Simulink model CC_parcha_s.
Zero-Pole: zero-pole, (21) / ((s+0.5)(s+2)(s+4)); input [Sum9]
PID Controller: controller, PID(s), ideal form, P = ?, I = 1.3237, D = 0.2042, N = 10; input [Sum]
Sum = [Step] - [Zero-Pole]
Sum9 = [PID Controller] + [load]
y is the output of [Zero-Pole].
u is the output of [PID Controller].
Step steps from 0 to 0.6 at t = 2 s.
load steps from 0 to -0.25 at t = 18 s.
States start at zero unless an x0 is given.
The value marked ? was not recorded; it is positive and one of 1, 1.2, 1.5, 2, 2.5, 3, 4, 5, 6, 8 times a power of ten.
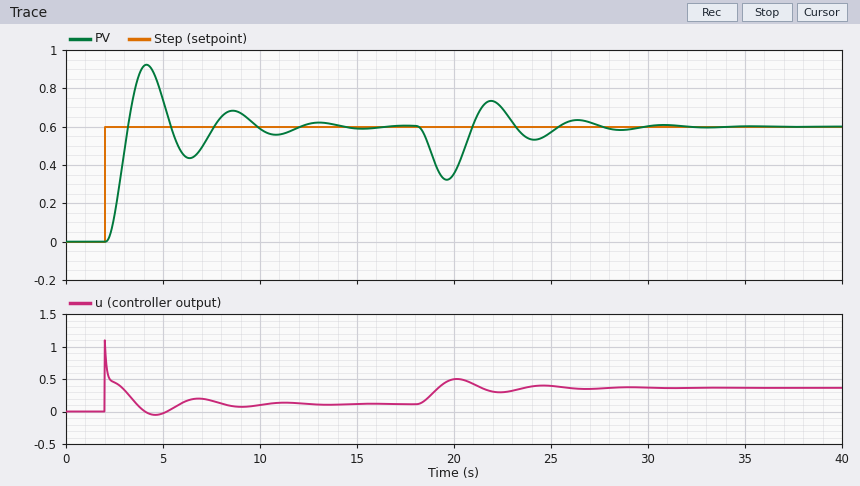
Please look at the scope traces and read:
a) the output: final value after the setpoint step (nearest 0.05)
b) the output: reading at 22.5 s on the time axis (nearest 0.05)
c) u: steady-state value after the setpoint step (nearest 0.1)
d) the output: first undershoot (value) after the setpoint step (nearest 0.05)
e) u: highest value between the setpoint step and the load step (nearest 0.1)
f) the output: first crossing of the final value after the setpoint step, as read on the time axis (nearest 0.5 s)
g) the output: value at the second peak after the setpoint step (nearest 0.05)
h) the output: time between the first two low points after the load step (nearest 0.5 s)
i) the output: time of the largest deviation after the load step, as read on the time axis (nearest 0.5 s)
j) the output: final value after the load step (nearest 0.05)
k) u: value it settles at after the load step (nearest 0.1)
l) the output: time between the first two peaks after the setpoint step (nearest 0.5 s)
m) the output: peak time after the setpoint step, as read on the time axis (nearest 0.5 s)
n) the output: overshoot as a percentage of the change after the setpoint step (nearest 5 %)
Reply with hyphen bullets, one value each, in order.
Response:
- 0.60
- 0.70
- 0.1
- 0.45
- 1.1
- 3.0 s
- 0.70
- 4.5 s
- 19.5 s
- 0.60
- 0.4
- 4.5 s
- 4.0 s
- 55 %
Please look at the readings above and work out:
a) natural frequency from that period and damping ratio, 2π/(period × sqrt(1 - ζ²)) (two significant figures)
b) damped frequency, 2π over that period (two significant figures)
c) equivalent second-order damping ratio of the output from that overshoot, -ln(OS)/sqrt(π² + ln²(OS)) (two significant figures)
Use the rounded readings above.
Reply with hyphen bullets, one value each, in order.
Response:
- 1.4 rad/s
- 1.4 rad/s
- 0.19
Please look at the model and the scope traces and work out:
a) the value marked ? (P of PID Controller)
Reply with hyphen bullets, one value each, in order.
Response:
- 0.6
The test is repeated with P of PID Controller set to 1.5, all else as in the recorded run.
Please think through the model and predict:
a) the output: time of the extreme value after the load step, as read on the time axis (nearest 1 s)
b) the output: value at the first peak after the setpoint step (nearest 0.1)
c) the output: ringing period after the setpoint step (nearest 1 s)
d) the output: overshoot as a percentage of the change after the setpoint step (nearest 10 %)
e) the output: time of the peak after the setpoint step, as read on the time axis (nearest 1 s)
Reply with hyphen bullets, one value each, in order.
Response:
- 19 s
- 1.0
- 3 s
- 70 %
- 3 s
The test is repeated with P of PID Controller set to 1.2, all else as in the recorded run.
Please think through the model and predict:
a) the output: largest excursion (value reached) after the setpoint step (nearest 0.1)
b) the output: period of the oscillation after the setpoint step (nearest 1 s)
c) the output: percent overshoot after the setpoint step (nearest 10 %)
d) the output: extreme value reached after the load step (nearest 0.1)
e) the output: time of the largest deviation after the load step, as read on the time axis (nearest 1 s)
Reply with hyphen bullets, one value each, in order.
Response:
- 1.0
- 3 s
- 70 %
- 0.4
- 19 s
